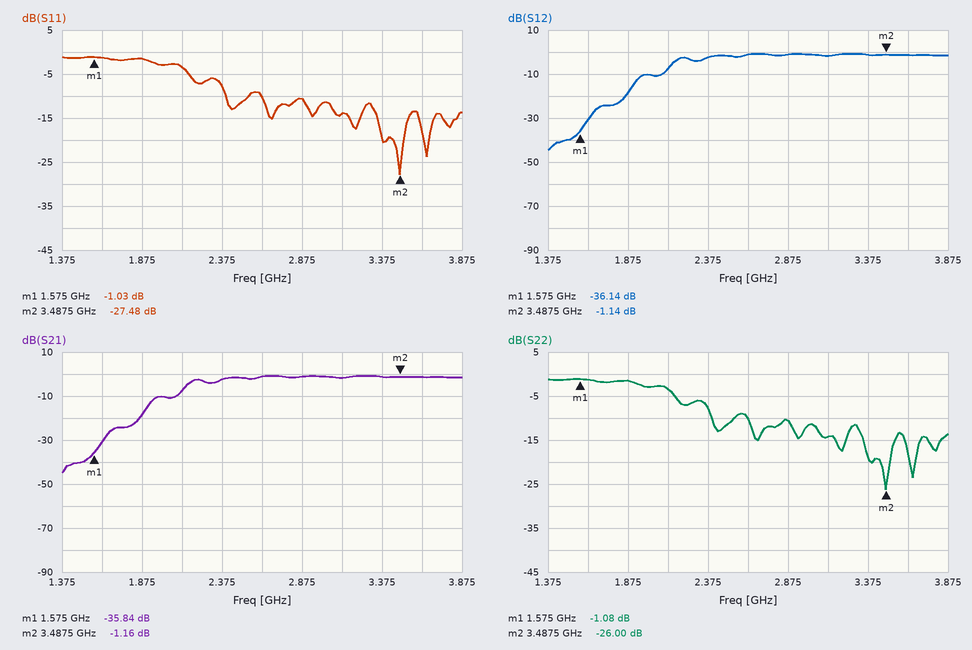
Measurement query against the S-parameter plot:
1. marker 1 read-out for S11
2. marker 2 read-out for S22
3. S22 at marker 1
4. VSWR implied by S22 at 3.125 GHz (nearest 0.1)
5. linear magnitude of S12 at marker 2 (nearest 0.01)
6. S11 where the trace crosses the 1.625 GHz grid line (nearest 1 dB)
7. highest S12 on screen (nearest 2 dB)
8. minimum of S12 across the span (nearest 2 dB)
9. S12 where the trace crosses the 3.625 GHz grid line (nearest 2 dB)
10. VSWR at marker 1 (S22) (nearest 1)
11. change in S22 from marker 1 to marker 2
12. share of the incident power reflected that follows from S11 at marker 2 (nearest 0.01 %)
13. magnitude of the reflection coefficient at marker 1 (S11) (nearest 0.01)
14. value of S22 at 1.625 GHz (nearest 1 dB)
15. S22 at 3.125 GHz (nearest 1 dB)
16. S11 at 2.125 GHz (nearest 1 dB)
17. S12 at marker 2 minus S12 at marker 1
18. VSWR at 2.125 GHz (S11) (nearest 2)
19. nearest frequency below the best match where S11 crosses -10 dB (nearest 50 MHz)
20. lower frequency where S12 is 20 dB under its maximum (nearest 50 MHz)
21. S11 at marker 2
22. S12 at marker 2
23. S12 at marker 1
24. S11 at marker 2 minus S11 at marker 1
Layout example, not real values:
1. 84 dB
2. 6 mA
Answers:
1. -1.03 dB
2. -26.00 dB
3. -1.08 dB
4. 1.5
5. 0.88
6. -1 dB
7. 0 dB
8. -44 dB
9. -2 dB
10. 16
11. -24.92 dB
12. 0.18 %
13. 0.89
14. -1 dB
15. -14 dB
16. -3 dB
17. 35.00 dB
18. 6
19. 2.60 GHz
20. 1.85 GHz
21. -27.48 dB
22. -1.14 dB
23. -36.14 dB
24. -26.45 dB
